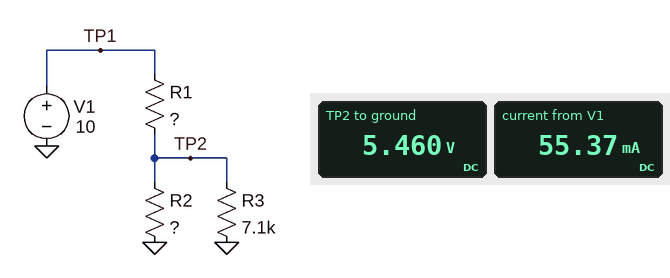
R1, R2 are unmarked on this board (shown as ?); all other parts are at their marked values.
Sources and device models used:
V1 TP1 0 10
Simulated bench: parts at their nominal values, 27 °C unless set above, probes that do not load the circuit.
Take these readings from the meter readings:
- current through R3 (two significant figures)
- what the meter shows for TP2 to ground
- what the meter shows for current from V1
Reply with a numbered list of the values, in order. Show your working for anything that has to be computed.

1. (5.46 V) / 7.1 kΩ = 770 µA
2. 5.460 V
3. 55.37 mA
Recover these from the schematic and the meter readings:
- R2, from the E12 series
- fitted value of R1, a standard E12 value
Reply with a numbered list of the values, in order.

1. 100 Ω
2. 82 Ω
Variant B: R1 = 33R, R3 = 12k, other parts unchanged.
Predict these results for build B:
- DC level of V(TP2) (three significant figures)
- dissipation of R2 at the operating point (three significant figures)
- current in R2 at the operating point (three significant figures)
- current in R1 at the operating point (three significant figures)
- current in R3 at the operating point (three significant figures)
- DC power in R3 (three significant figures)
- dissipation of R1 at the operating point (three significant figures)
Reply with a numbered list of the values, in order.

1. 7.50 V
2. 563 mW
3. 75.0 mA
4. 75.7 mA
5. 625 µA
6. 4.69 mW
7. 189 mW
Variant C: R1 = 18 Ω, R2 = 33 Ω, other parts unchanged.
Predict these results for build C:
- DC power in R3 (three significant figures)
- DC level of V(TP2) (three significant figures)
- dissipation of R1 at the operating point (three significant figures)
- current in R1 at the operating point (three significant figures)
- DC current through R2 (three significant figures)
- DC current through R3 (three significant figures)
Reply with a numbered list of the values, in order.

1. 5.88 mW
2. 6.46 V
3. 696 mW
4. 197 mA
5. 196 mA
6. 910 µA
